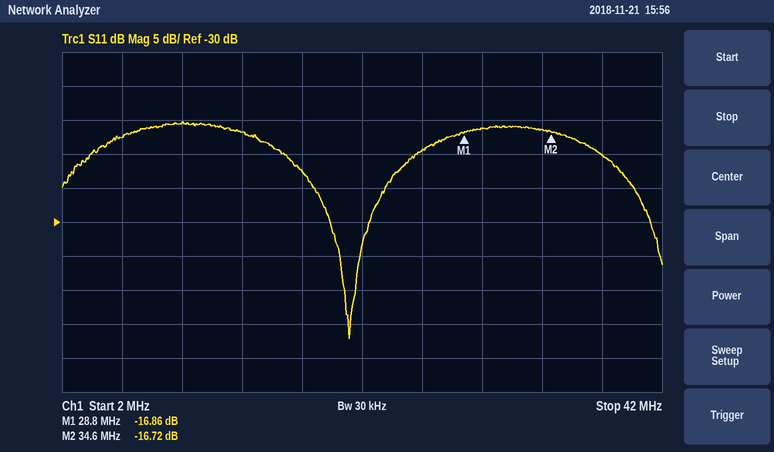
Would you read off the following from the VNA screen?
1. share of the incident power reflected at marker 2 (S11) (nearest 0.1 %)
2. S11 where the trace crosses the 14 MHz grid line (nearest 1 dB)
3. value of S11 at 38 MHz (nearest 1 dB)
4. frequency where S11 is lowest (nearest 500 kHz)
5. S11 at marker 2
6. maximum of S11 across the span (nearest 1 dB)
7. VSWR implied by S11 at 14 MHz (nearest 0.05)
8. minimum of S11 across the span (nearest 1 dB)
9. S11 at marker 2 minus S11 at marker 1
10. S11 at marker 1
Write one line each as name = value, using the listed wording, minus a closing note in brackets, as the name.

share of the incident power reflected at marker 2 (S11) = 2.1 %
S11 where the trace crosses the 14 MHz grid line = -17 dB
value of S11 at 38 MHz = -20 dB
frequency where S11 is lowest = 21.0 MHz
S11 at marker 2 = -16.72 dB
maximum of S11 across the span = -15 dB
VSWR implied by S11 at 14 MHz = 1.35
minimum of S11 across the span = -47 dB
S11 at marker 2 minus S11 at marker 1 = 0.14 dB
S11 at marker 1 = -16.86 dB
